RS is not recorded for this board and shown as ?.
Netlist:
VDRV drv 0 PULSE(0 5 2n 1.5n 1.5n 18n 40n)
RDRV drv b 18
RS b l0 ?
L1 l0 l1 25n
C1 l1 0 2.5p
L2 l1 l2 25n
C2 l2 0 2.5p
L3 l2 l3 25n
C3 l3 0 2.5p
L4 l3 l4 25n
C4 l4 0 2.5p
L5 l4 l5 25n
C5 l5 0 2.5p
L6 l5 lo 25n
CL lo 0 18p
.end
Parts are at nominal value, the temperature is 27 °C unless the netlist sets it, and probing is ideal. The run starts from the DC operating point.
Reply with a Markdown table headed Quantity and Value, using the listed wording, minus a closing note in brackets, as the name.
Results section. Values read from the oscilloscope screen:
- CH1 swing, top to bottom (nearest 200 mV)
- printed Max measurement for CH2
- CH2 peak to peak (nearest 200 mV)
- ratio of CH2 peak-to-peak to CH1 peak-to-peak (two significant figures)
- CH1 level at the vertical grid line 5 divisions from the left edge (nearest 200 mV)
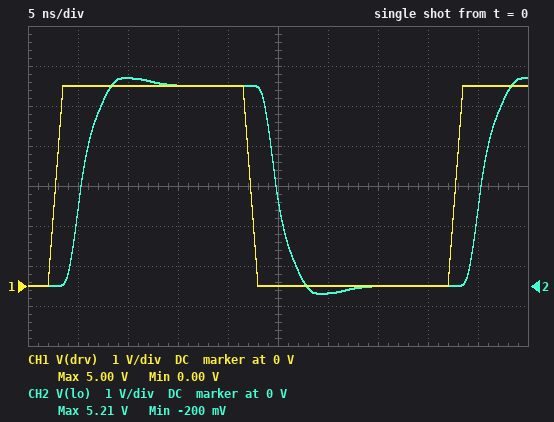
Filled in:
| Quantity | Value |
|---|---|
| CH1 swing, top to bottom | 5.0 V |
| printed Max measurement for CH2 | 5.21 V |
| CH2 peak to peak | 5.4 V |
| ratio of CH2 peak-to-peak to CH1 peak-to-peak | 1.1 |
| CH1 level at the vertical grid line 5 divisions from the left edge | 0 V |
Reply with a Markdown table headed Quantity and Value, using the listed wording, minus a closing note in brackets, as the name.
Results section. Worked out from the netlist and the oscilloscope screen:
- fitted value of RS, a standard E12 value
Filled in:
| Quantity | Value |
|---|---|
| fitted value of RS, a standard E12 value | 68 Ω |
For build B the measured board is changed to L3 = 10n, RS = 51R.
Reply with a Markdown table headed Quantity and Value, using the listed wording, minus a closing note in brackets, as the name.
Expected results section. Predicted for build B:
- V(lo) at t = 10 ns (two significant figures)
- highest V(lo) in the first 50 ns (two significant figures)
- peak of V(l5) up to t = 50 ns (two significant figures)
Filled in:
| Quantity | Value |
|---|---|
| V(lo) at t = 10 ns | 5.4 V |
| highest V(lo) in the first 50 ns | 5.6 V |
| peak of V(l5) up to t = 50 ns | 5.5 V |
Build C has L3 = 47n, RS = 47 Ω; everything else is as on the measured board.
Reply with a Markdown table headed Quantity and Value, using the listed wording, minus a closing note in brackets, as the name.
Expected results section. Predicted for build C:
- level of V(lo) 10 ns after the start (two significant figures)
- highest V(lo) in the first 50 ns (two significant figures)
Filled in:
| Quantity | Value |
|---|---|
| level of V(lo) 10 ns after the start | 5.9 V |
| highest V(lo) in the first 50 ns | 6.0 V |
